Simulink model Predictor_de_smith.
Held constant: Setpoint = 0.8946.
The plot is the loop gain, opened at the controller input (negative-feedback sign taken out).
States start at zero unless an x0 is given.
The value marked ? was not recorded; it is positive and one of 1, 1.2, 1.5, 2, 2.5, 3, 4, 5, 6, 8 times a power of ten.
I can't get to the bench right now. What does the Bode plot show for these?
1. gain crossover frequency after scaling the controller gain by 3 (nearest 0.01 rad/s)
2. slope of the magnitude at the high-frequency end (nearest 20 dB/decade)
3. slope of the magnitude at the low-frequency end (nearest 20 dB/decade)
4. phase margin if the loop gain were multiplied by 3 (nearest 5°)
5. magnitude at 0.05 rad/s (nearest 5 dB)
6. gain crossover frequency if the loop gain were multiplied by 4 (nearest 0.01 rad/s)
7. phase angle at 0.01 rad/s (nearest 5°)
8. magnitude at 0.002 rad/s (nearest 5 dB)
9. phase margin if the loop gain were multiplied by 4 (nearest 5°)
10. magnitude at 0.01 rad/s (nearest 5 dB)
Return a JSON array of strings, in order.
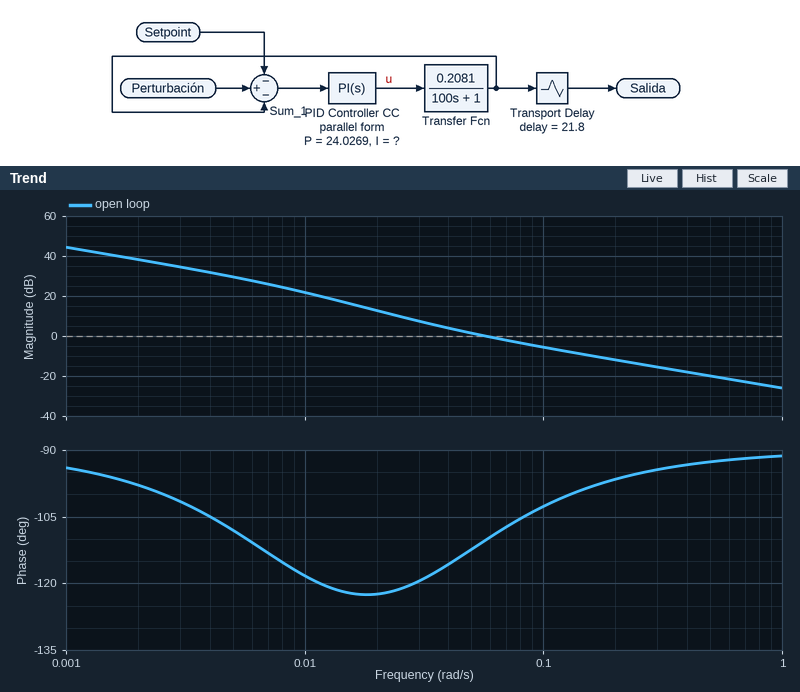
["0.15 rad/s", "-20 dB/decade", "-20 dB/decade", "80°", "0 dB", "0.20 rad/s", "-120°", "40 dB", "85°", "20 dB"]
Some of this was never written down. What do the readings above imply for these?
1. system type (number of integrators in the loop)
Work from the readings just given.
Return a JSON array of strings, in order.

["1"]
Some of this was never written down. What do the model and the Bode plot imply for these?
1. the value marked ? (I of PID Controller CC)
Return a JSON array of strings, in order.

["0.8"]
